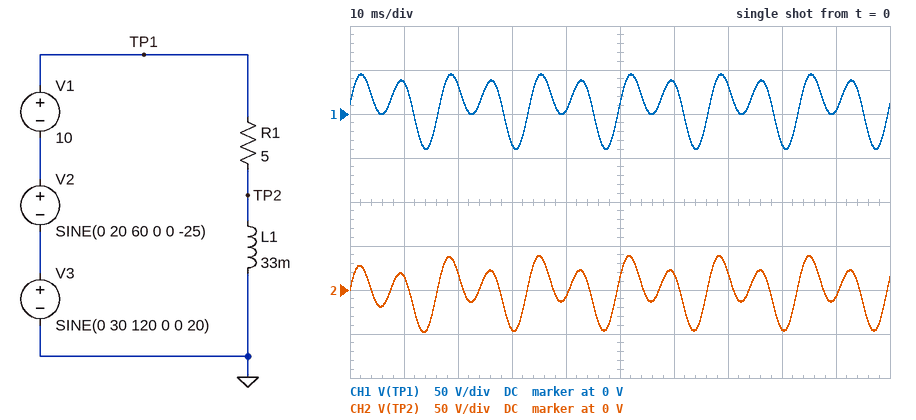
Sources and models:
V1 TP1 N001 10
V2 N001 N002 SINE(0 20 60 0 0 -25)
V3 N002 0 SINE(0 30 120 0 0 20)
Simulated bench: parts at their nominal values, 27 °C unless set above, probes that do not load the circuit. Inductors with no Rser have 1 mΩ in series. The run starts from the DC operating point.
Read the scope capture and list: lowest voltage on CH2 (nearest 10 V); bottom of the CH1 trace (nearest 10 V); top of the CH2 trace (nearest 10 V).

-50 V
-40 V
40 V
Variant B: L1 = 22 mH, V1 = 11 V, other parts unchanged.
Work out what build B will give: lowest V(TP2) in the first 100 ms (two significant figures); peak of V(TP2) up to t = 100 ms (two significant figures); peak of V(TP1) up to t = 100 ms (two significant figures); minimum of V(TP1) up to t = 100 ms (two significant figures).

-44 V
39 V
46 V
-39 V
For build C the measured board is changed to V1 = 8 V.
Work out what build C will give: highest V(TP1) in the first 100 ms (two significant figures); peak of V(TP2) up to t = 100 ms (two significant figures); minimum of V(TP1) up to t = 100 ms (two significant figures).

43 V
39 V
-42 V
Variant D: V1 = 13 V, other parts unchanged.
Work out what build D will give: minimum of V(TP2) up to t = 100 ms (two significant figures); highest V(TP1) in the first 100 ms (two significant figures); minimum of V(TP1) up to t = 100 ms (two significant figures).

-48 V
48 V
-37 V
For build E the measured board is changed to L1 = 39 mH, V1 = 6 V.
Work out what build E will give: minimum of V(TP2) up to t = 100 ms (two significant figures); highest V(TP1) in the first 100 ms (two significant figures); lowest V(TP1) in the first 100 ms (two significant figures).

-49 V
41 V
-44 V
